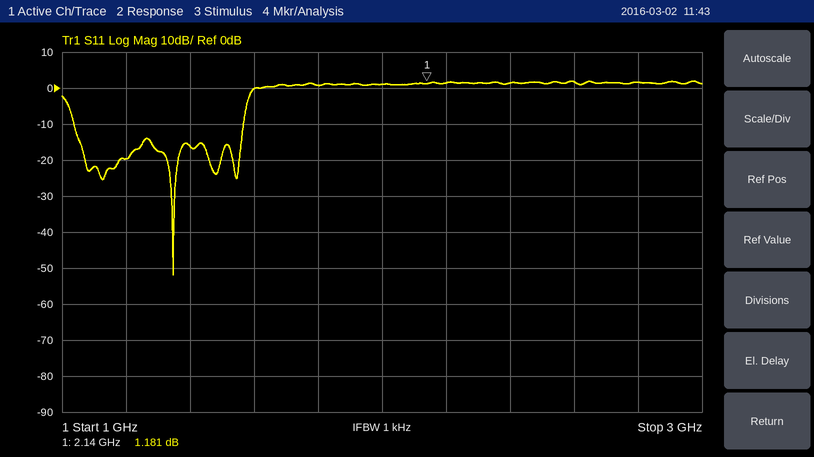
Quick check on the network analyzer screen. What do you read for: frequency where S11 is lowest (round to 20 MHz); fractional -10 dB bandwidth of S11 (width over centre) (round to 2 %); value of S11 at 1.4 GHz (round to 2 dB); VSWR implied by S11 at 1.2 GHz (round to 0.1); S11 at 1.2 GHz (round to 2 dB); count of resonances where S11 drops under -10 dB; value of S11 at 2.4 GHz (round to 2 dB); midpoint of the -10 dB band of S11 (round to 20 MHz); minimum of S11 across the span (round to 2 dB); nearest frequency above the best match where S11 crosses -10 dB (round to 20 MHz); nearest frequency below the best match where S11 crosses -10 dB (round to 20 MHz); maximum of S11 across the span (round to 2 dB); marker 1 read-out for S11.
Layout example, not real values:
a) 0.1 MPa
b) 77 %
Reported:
a) 1.34 GHz
b) 40 %
c) -16 dB
d) 1.2
e) -20 dB
f) 4
g) 2 dB
h) 1.30 GHz
i) -52 dB
j) 1.56 GHz
k) 1.04 GHz
l) 2 dB
m) 1.181 dB
